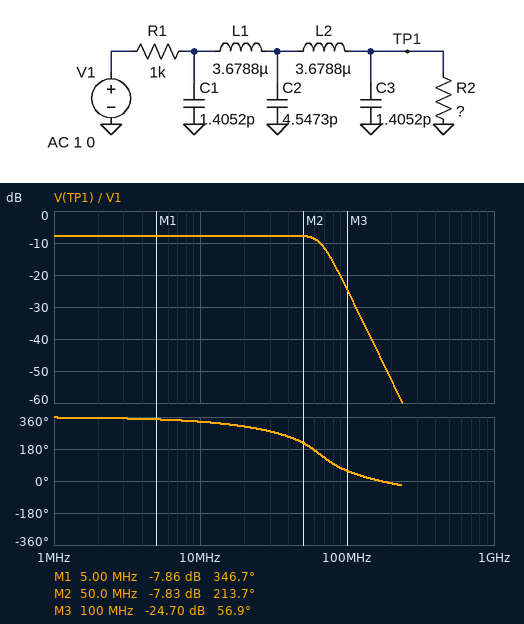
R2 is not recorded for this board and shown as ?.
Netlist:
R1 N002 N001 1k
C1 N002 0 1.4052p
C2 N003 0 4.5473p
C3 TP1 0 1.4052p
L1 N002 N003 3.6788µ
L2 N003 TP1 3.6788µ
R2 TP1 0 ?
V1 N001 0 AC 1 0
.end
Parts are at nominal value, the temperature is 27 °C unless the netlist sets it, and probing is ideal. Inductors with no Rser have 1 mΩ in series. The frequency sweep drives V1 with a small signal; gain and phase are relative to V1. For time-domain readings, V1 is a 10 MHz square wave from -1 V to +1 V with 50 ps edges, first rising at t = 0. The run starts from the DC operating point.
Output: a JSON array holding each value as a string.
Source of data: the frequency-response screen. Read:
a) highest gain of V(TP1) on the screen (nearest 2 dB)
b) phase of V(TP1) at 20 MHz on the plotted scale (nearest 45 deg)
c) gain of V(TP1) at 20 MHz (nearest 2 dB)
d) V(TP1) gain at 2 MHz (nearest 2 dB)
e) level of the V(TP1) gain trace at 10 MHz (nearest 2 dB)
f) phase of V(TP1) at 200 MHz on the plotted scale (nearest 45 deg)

["-8 dB", "315 deg", "-8 dB", "-8 dB", "-8 dB", "0 deg"]
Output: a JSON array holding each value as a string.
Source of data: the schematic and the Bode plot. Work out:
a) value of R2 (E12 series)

["680 Ω"]
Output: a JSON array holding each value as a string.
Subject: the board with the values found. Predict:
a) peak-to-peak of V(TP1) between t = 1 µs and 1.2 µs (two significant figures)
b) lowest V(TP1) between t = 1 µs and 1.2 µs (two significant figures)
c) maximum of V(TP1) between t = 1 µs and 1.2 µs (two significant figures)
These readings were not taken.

["1.0 V", "-510 mV", "510 mV"]
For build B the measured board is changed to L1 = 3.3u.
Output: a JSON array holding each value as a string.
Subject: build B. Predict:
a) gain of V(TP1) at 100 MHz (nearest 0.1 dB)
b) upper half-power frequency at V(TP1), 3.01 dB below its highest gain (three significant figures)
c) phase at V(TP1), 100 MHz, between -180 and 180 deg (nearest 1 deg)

["-23.4 dB", "69.2 MHz", "61 deg"]
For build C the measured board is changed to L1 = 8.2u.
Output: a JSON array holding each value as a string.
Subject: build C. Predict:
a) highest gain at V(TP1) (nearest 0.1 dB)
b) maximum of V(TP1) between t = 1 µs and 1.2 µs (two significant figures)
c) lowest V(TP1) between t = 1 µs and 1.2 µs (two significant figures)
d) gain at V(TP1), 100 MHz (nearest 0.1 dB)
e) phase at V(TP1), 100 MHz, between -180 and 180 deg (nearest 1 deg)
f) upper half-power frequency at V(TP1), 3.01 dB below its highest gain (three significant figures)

["-7.9 dB", "450 mV", "-450 mV", "-33.7 dB", "42 deg", "52.6 MHz"]
